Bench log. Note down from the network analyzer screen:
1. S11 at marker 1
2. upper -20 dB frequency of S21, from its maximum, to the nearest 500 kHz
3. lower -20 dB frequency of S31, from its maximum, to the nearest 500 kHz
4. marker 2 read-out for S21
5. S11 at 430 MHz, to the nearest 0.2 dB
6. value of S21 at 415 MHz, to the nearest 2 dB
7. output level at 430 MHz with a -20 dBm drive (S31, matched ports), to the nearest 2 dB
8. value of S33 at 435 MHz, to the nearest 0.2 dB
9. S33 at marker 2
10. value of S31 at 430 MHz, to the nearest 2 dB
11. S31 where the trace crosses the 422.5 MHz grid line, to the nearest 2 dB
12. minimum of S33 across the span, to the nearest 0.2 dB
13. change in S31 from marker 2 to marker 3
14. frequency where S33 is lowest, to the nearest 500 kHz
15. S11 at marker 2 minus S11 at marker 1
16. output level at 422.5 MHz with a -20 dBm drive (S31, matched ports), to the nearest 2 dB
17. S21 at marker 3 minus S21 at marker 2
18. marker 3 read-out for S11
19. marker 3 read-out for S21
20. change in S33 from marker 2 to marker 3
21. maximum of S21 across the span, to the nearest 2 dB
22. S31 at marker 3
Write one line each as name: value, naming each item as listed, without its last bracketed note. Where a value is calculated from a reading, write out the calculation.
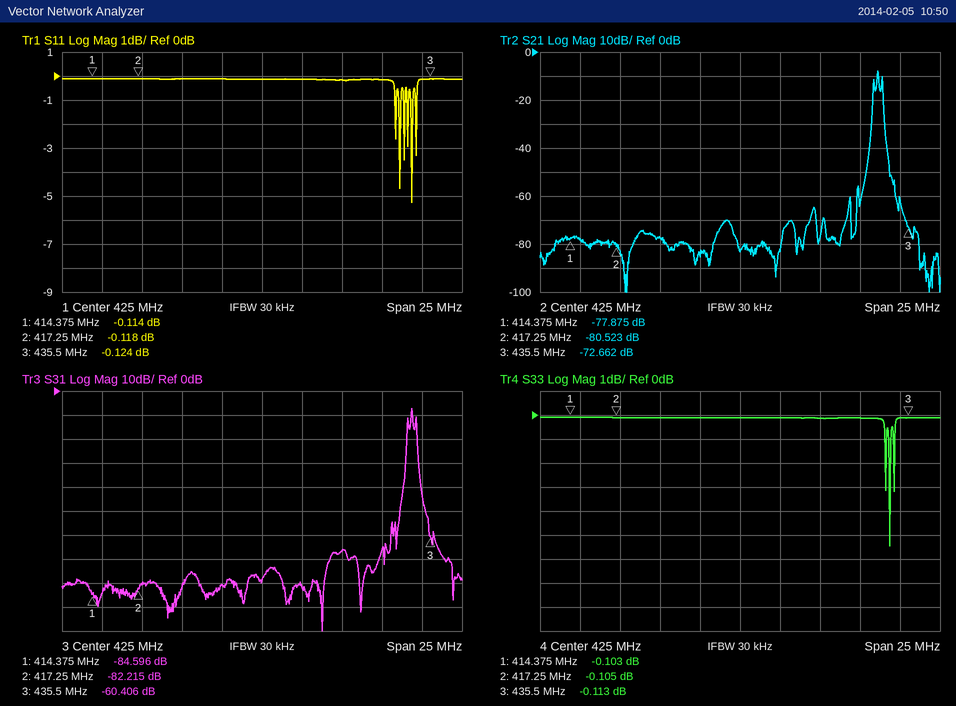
S11 at marker 1: -0.114 dB
upper -20 dB frequency of S21, from its maximum, to the nearest 500 kHz: 434.0 MHz
lower -20 dB frequency of S31, from its maximum, to the nearest 500 kHz: 434.0 MHz
marker 2 read-out for S21: -80.523 dB
S11 at 430 MHz, to the nearest 0.2 dB: -0.2 dB
value of S21 at 415 MHz, to the nearest 2 dB: -78 dB
output level at 430 MHz with a -20 dBm drive (S31, matched ports), to the nearest 2 dB: -20 dBm + (-66 dB) = -86 dBm
value of S33 at 435 MHz, to the nearest 0.2 dB: -0.2 dB
S33 at marker 2: -0.105 dB
value of S31 at 430 MHz, to the nearest 2 dB: -66 dB
S31 where the trace crosses the 422.5 MHz grid line, to the nearest 2 dB: -80 dB
minimum of S33 across the span, to the nearest 0.2 dB: -5.4 dB
change in S31 from marker 2 to marker 3: -60.406 − (-82.215) = 21.809 dB
frequency where S33 is lowest, to the nearest 500 kHz: 434.5 MHz
S11 at marker 2 minus S11 at marker 1: -0.118 − (-0.114) = -0.004 dB
output level at 422.5 MHz with a -20 dBm drive (S31, matched ports), to the nearest 2 dB: -20 dBm + (-80 dB) = -100 dBm
S21 at marker 3 minus S21 at marker 2: -72.662 − (-80.523) = 7.861 dB
marker 3 read-out for S11: -0.124 dB
marker 3 read-out for S21: -72.662 dB
change in S33 from marker 2 to marker 3: -0.113 − (-0.105) = -0.008 dB
maximum of S21 across the span, to the nearest 2 dB: -8 dB
S31 at marker 3: -60.406 dB
